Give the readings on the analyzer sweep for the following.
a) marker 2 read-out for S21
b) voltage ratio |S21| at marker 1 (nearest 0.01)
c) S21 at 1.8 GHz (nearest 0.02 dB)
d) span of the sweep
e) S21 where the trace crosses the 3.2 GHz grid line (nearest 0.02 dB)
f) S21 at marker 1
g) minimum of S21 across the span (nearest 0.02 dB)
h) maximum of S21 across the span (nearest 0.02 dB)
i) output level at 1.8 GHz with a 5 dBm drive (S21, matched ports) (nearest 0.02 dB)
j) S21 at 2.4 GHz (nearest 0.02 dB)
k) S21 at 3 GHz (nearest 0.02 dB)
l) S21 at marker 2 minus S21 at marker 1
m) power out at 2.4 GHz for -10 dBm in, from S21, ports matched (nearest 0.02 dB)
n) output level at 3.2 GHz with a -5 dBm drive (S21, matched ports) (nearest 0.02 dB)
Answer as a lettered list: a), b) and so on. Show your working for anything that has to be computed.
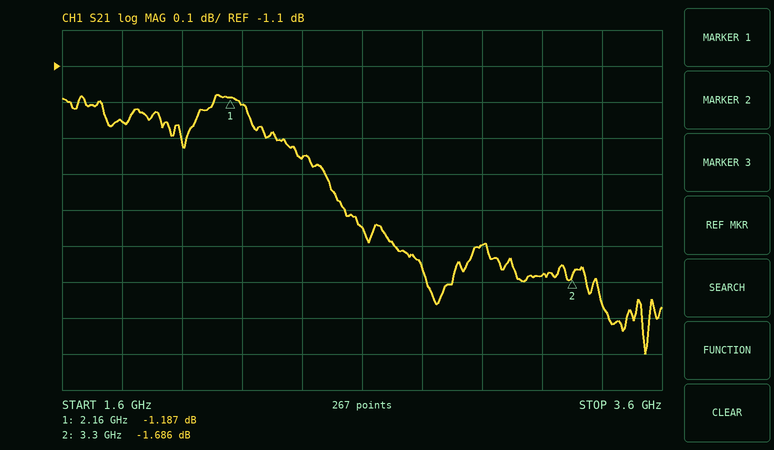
a) -1.686 dB
b) 10^(-1.187/20) ≈ 0.87
c) -1.26 dB
d) 2 GHz
e) -1.68 dB
f) -1.187 dB
g) -1.90 dB
h) -1.18 dB
i) 5 dBm + (-1.26 dB) = 3.74 dBm
j) -1.36 dB
k) -1.60 dB
l) -1.686 − (-1.187) = -0.499 dB
m) -10 dBm + (-1.36 dB) = -11.36 dBm
n) -5 dBm + (-1.68 dB) = -6.68 dBm
